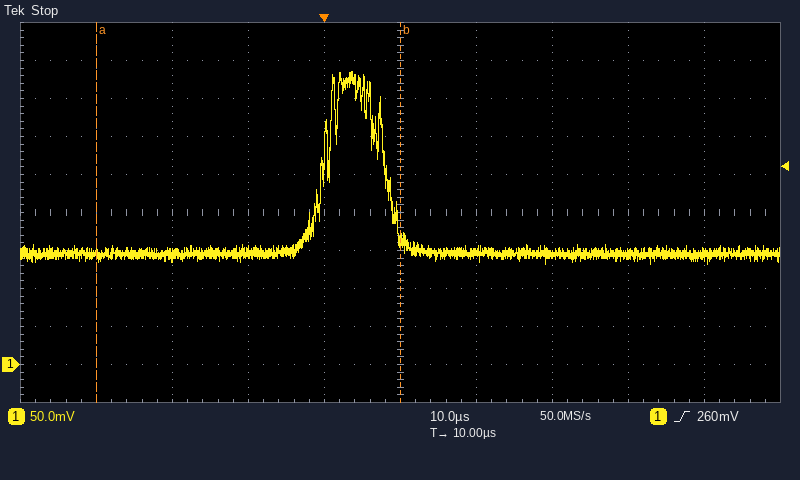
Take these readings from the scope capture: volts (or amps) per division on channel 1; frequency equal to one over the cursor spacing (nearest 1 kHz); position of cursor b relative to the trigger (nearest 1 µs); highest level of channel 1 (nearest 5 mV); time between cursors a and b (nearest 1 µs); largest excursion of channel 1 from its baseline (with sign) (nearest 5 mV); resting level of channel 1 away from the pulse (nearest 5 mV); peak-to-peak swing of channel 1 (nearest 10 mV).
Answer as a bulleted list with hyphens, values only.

- 50 mV
- 25 kHz
- +10 µs
- 385 mV
- 40 µs
- +240 mV
- 145 mV
- 250 mV
